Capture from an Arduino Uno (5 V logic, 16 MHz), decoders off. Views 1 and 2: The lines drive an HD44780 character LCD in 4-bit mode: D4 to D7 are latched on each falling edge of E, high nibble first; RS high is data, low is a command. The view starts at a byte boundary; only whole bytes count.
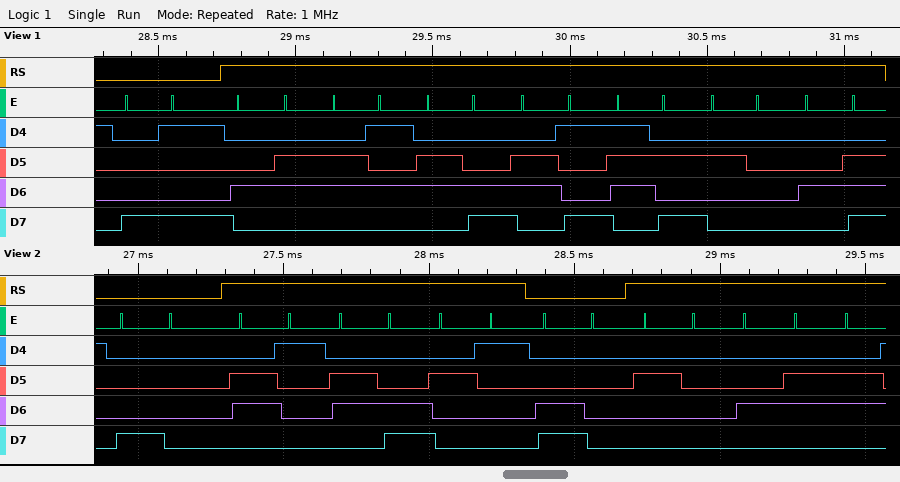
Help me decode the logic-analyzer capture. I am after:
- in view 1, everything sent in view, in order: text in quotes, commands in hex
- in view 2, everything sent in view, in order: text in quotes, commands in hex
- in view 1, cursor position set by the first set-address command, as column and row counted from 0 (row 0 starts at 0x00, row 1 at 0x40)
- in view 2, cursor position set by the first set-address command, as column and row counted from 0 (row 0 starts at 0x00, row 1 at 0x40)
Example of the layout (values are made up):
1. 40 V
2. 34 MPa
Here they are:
1. 0x89 "Feliz N"
2. 0x80 "al!" 0xC0 " F"
3. column 9, row 0
4. column 0, row 0
